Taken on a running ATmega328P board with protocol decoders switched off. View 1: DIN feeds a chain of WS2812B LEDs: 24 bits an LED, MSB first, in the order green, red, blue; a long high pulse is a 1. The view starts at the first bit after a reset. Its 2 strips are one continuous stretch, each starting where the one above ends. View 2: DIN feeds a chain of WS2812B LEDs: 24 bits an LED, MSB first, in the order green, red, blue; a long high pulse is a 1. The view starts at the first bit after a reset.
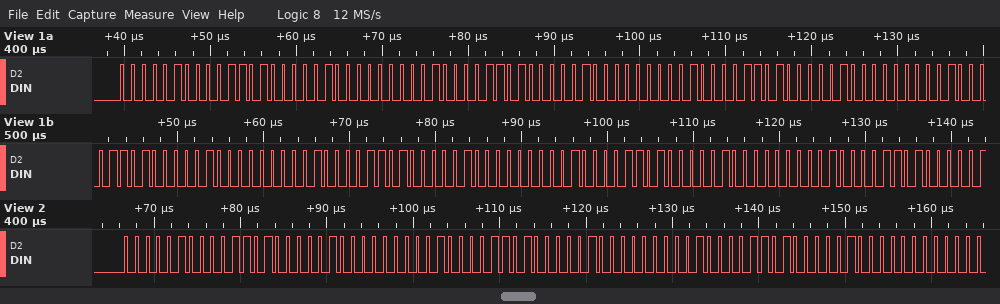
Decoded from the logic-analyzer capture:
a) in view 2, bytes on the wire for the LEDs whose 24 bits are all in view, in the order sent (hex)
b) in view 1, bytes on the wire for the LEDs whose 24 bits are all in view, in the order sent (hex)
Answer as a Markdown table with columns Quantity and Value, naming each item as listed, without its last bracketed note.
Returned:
| Quantity | Value |
|---|---|
| in view 2, bytes on the wire for the LEDs whose 24 bits are all in view, in the order sent | 04 34 10 04 34 10 04 34 10 |
| in view 1, bytes on the wire for the LEDs whose 24 bits are all in view, in the order sent | 04 34 10 04 34 10 04 34 10 04 34 10 04 34 10 04 34 10 |
